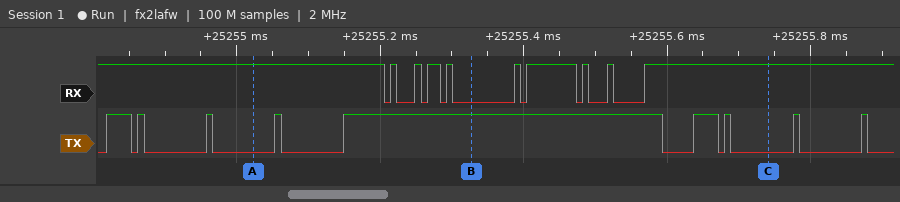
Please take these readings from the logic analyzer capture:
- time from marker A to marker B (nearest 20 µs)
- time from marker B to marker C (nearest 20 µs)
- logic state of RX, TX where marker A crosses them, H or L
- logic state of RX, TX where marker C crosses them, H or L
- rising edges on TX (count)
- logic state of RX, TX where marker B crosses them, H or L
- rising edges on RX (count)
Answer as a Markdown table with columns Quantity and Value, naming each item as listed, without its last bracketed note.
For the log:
| Quantity | Value |
|---|---|
| time from marker A to marker B | 300 µs |
| time from marker B to marker C | 420 µs |
| logic state of RX, TX where marker A crosses them, H or L | RX=H, TX=L |
| logic state of RX, TX where marker C crosses them, H or L | RX=H, TX=L |
| rising edges on TX | 9 |
| logic state of RX, TX where marker B crosses them, H or L | RX=L, TX=H |
| rising edges on RX | 9 |
